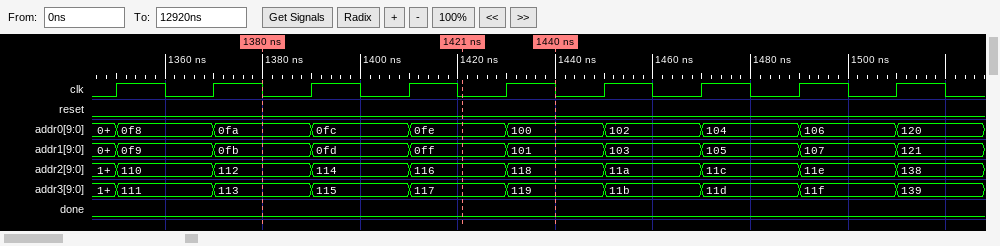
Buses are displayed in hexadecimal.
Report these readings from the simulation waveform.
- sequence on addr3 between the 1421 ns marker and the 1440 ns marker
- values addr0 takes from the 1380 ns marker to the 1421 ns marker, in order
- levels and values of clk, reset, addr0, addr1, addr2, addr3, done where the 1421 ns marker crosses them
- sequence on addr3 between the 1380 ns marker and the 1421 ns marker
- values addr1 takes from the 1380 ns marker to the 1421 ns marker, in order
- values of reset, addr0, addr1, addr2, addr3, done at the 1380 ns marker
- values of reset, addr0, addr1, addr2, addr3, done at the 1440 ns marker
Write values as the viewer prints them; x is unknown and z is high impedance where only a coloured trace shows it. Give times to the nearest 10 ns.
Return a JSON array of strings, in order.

["117, 119", "0fa, 0fc, 0fe", "clk=0, reset=0, addr0=0fe, addr1=0ff, addr2=116, addr3=117, done=0", "113, 115, 117", "0fb, 0fd, 0ff", "reset=0, addr0=0fa, addr1=0fb, addr2=112, addr3=113, done=0", "reset=0, addr0=100, addr1=101, addr2=118, addr3=119, done=0"]
